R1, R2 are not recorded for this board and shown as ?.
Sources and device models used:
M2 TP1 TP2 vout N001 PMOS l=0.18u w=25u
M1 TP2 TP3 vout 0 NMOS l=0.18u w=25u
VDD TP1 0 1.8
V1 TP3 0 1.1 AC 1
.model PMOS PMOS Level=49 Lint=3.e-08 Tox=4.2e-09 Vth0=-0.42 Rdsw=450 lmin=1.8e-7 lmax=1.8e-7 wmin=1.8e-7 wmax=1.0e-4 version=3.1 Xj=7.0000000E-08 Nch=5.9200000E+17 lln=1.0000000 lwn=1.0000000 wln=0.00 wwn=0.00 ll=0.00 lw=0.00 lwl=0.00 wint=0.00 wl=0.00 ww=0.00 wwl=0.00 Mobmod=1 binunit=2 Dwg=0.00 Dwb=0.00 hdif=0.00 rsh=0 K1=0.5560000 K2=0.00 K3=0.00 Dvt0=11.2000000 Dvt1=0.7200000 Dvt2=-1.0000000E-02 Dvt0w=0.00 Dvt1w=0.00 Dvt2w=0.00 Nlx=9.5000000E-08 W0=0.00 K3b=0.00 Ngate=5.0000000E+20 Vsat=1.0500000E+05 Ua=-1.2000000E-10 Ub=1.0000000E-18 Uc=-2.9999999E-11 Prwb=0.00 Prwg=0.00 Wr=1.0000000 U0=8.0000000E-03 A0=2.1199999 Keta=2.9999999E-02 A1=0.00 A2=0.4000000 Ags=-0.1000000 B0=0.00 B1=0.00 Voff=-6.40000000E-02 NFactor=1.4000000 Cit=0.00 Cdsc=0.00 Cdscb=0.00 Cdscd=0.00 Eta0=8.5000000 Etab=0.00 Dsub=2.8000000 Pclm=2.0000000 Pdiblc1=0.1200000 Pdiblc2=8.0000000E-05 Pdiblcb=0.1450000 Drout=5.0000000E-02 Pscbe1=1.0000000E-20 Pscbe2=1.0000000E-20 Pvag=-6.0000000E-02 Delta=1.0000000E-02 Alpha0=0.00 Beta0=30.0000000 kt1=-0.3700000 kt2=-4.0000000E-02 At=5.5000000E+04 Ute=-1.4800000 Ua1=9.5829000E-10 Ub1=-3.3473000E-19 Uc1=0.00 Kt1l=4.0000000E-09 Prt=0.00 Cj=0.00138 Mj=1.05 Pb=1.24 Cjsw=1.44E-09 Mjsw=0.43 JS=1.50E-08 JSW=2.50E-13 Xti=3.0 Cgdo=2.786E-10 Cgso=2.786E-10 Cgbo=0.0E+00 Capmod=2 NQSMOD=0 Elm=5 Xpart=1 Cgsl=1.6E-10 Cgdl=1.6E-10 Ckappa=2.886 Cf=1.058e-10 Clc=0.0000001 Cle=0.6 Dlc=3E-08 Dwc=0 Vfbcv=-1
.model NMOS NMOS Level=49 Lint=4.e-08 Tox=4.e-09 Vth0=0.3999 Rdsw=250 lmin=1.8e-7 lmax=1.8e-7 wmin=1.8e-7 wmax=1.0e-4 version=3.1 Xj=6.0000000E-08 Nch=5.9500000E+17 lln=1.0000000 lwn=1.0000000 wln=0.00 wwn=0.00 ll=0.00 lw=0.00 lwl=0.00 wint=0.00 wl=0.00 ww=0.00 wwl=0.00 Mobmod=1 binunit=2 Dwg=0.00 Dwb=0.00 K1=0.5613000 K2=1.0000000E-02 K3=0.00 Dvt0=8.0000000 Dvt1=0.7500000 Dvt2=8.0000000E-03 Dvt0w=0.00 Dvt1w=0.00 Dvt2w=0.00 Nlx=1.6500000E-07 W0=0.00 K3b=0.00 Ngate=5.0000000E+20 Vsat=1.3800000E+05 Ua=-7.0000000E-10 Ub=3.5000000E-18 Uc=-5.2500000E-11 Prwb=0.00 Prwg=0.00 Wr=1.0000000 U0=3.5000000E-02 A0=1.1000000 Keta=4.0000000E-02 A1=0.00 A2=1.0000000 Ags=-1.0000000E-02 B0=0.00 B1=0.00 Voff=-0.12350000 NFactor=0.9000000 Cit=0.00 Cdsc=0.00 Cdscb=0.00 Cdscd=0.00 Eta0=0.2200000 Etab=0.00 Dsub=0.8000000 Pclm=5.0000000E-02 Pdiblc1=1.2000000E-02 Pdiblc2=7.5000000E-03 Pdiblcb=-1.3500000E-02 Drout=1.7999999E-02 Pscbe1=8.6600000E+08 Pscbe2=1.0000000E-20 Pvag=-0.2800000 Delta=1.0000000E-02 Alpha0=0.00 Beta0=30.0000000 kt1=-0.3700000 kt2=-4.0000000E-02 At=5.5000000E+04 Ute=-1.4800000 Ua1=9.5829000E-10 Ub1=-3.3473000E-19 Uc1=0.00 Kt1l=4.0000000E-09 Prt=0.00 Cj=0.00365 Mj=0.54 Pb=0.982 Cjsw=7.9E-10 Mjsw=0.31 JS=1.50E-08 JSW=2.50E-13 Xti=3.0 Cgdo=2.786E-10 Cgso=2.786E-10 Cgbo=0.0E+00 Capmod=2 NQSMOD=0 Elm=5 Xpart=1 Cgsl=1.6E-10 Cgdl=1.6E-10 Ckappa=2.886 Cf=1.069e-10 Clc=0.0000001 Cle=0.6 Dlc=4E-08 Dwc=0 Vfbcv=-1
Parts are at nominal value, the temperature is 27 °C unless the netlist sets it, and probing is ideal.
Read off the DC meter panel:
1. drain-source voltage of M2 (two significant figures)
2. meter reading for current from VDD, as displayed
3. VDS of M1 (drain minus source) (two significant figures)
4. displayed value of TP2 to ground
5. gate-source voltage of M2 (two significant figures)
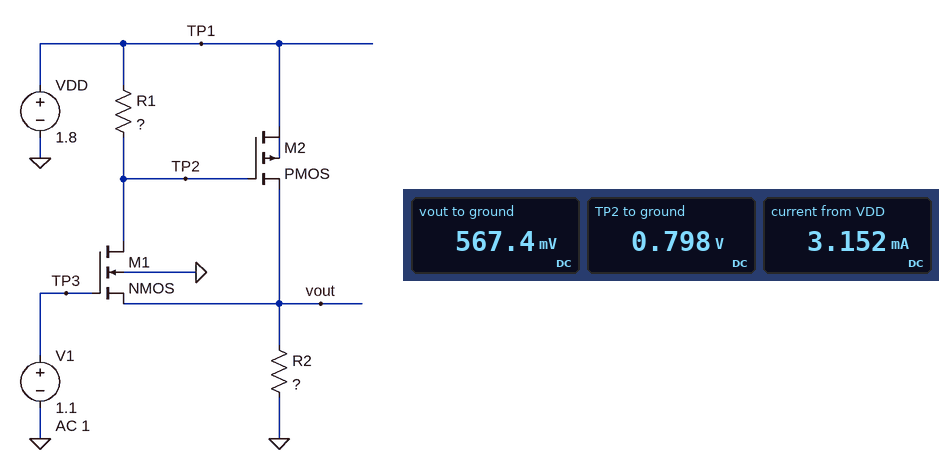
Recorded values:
1.2 V
3.152 mA
230 mV
0.798 V
230 mV
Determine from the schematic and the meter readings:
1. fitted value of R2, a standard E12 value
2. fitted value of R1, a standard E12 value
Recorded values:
180 Ω
6.8 kΩ
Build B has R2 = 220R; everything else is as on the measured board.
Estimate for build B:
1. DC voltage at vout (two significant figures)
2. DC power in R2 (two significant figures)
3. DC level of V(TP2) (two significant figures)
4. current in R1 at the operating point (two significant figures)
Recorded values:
580 mV
1.5 mW
890 mV
130 µA
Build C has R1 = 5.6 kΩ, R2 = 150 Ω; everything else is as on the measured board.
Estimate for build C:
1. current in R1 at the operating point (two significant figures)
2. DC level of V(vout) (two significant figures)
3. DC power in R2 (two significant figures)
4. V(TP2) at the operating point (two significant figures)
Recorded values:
190 µA
550 mV
2.0 mW
720 mV
